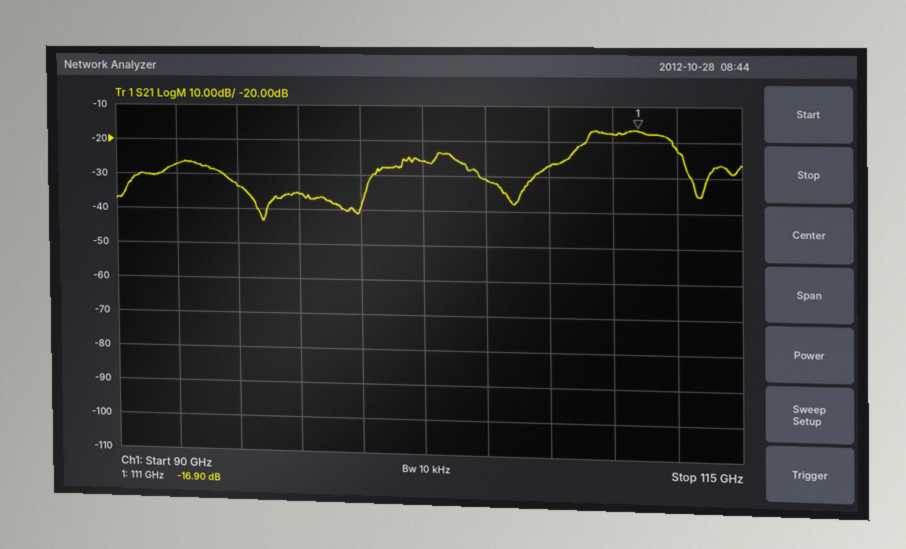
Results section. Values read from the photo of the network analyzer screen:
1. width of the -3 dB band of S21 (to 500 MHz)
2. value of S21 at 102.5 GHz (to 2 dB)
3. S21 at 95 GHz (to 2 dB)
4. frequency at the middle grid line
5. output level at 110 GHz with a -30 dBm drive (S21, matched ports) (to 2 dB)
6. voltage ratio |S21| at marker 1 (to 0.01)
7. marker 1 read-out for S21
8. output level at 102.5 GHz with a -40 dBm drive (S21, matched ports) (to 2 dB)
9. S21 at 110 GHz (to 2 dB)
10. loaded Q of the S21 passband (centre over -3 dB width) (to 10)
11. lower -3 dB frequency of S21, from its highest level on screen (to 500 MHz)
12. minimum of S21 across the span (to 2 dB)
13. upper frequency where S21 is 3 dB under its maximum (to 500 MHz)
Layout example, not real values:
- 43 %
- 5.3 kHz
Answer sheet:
- 3.5 GHz
- -26 dB
- -34 dB
- 102.5 GHz
- -48 dBm
- 0.14
- -16.90 dB
- -66 dBm
- -18 dB
- 30
- 109.0 GHz
- -44 dB
- 112.5 GHz
